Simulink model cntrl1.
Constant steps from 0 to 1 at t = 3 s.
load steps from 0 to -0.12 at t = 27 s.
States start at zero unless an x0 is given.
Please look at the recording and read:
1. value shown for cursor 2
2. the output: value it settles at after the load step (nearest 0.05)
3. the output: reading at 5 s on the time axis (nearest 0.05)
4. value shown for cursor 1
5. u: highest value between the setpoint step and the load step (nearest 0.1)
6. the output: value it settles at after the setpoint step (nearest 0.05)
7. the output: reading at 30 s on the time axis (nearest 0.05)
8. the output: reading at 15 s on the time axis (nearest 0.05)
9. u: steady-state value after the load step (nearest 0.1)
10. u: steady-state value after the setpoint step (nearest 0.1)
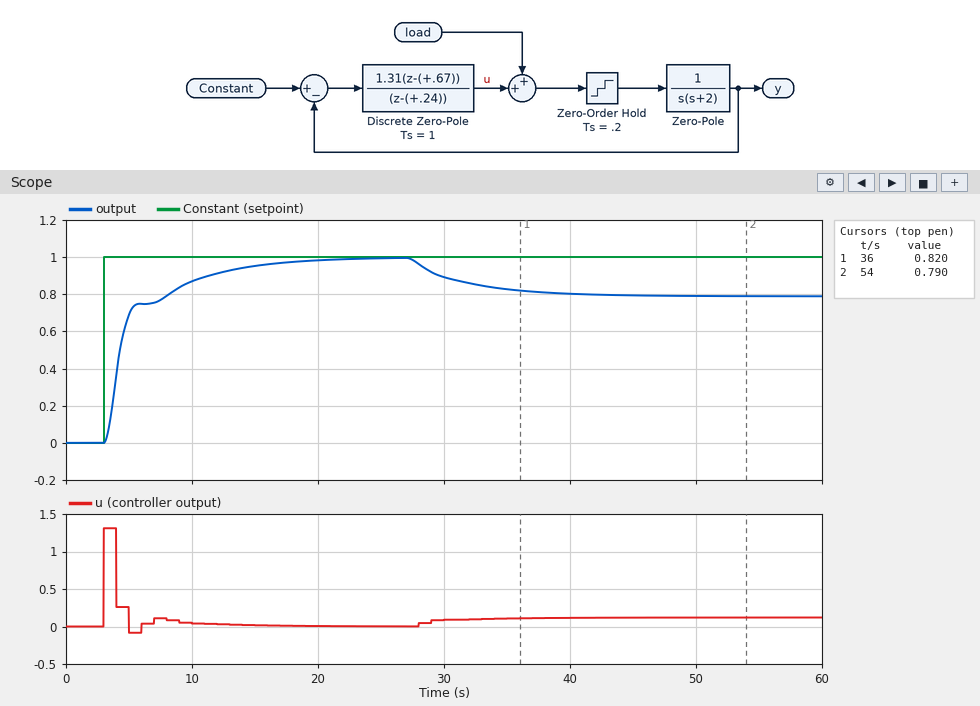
0.790
0.80
0.70
0.820
1.3
1.00
0.90
0.95
0.1
0.0
